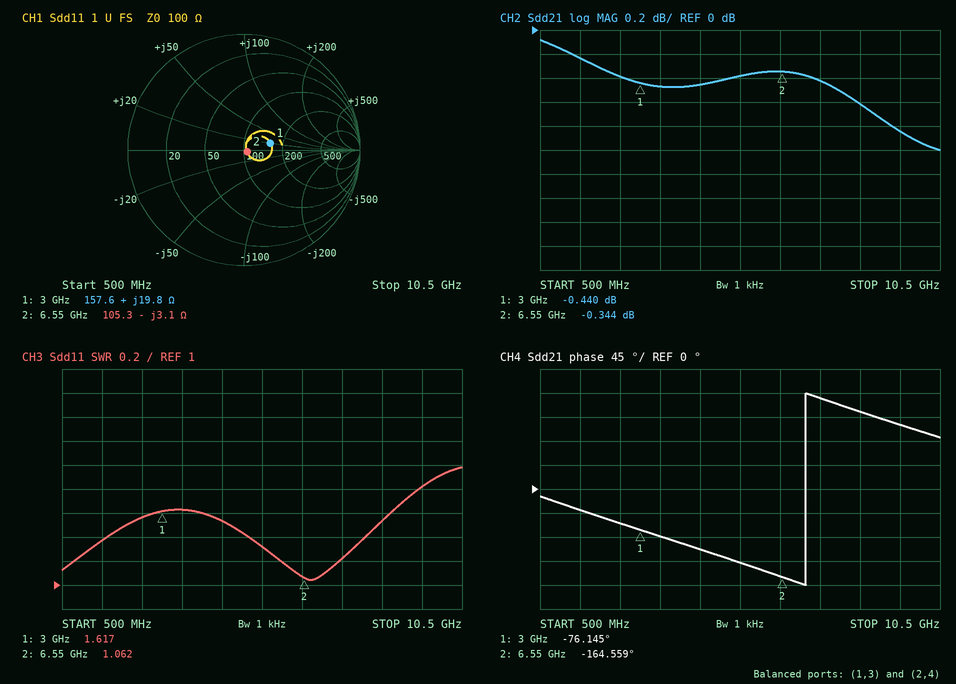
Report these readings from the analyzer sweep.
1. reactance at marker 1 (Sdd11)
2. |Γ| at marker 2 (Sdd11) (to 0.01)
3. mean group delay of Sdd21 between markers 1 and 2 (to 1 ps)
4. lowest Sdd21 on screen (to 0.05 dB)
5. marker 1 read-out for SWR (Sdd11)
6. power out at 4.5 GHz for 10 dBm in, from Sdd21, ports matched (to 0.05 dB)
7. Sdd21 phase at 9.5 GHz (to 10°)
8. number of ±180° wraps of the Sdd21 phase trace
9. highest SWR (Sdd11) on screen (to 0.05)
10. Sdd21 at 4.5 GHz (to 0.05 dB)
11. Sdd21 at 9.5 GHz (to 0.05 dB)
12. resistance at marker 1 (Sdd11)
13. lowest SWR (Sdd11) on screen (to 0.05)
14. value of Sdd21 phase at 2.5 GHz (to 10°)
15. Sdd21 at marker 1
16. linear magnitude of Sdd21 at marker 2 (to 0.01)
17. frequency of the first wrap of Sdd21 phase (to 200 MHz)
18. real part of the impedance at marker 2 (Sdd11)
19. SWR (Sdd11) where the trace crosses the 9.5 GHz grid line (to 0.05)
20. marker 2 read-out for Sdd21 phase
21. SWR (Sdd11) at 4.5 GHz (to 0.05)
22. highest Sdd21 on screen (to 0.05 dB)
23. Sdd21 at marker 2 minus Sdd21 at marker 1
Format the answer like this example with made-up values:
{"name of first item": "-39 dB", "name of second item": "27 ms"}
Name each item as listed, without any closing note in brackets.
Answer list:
{"reactance at marker 1": "+19.8 Ω", "|Γ| at marker 2 (Sdd11)": "0.03", "mean group delay of Sdd21 between markers 1 and 2": "69 ps", "lowest Sdd21 on screen": "-1.00 dB", "marker 1 read-out for SWR": "1.617", "power out at 4.5 GHz for 10 dBm in, from Sdd21, ports matched": "9.55 dBm", "Sdd21 phase at 9.5 GHz": "120°", "number of ±180° wraps of the Sdd21 phase trace": "1", "highest SWR (Sdd11) on screen": "2.00", "Sdd21 at 4.5 GHz": "-0.45 dB", "Sdd21 at 9.5 GHz": "-0.85 dB", "resistance at marker 1": "157.6 Ω", "lowest SWR (Sdd11) on screen": "1.05", "value of Sdd21 phase at 2.5 GHz": "-60°", "Sdd21 at marker 1": "-0.440 dB", "linear magnitude of Sdd21 at marker 2": "0.96", "frequency of the first wrap of Sdd21 phase": "7.2 GHz", "real part of the impedance at marker 2": "105.3 Ω", "SWR (Sdd11) where the trace crosses the 9.5 GHz grid line": "1.80", "marker 2 read-out for Sdd21 phase": "-164.559°", "SWR (Sdd11) at 4.5 GHz": "1.55", "highest Sdd21 on screen": "-0.10 dB", "Sdd21 at marker 2 minus Sdd21 at marker 1": "0.096 dB"}
